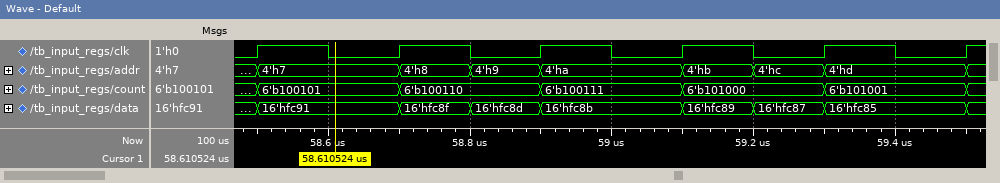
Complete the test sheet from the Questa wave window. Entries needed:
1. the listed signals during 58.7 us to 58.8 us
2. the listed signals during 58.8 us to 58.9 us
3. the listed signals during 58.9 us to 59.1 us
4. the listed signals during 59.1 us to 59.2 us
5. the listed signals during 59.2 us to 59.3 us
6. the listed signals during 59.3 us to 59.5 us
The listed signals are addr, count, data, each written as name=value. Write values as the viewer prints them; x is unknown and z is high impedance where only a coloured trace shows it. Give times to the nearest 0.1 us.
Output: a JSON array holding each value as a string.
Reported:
["addr=4'h8, count=6'b100110, data=16'hfc8f", "addr=4'h9, count=6'b100110, data=16'hfc8d", "addr=4'ha, count=6'b100111, data=16'hfc8b", "addr=4'hb, count=6'b101000, data=16'hfc89", "addr=4'hc, count=6'b101000, data=16'hfc87", "addr=4'hd, count=6'b101001, data=16'hfc85"]
